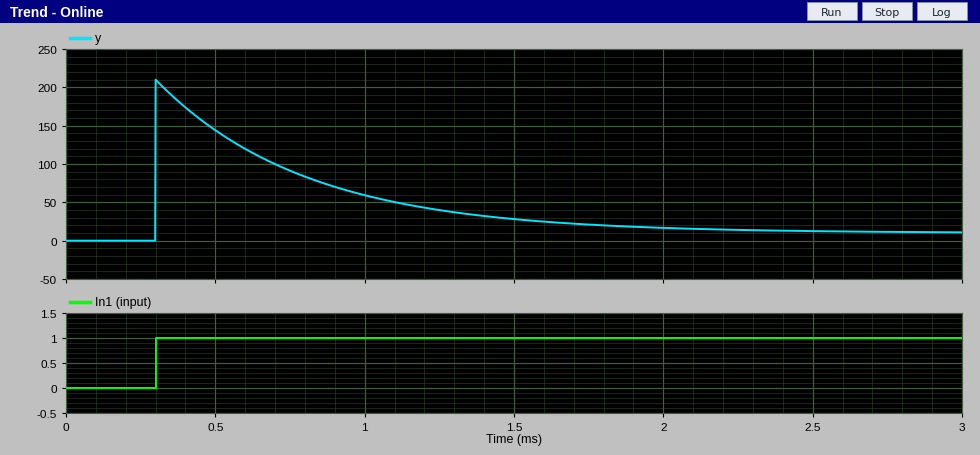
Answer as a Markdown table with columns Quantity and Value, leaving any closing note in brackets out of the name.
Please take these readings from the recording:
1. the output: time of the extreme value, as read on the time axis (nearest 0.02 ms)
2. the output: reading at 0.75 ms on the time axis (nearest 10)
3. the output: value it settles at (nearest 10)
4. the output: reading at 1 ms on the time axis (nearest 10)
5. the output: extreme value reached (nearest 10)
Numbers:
| Quantity | Value |
|---|---|
| the output: time of the extreme value, as read on the time axis | 0.30 ms |
| the output: reading at 0.75 ms on the time axis | 90 |
| the output: value it settles at | 10 |
| the output: reading at 1 ms on the time axis | 60 |
| the output: extreme value reached | 210 |
